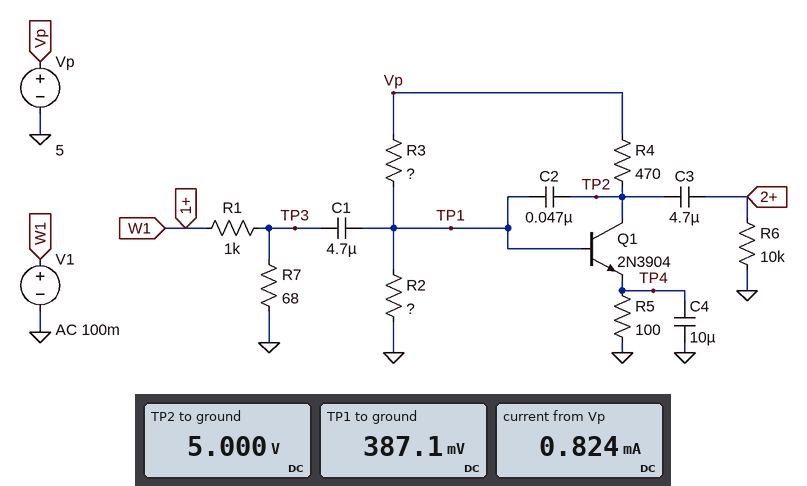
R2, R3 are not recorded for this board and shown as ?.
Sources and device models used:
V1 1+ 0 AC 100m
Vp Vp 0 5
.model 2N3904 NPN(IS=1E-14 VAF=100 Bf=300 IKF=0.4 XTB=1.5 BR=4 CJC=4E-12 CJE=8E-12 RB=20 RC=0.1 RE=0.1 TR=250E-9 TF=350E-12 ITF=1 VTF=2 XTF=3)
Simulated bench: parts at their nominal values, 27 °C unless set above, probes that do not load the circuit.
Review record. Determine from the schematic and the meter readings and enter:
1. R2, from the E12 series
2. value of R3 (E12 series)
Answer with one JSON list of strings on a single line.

["470 Ω", "5.6 kΩ"]
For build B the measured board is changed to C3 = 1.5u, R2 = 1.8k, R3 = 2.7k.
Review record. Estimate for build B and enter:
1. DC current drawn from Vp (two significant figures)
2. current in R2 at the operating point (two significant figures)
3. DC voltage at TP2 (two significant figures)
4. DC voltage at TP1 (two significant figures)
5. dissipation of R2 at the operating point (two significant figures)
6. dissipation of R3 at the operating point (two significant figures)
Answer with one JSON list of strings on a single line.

["9.9 mA", "900 µA", "950 mV", "1.6 V", "1.5 mW", "4.2 mW"]
